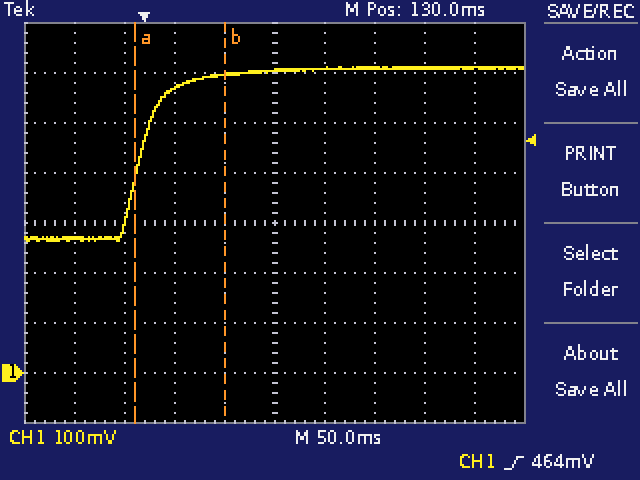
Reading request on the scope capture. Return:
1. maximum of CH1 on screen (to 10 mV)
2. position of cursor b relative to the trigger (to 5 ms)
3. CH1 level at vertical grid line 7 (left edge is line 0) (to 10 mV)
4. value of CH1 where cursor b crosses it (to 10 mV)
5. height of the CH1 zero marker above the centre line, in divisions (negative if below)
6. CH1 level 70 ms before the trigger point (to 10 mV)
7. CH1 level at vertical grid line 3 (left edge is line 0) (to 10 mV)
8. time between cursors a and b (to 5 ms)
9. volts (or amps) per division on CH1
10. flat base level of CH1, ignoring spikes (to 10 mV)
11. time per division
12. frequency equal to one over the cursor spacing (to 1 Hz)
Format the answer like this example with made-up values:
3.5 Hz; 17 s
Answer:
610 mV; +80 ms; 610 mV; 600 mV; -3.0 div; 270 mV; 570 mV; 90 ms; 100 mV; 270 mV; 50 ms; 11 Hz
